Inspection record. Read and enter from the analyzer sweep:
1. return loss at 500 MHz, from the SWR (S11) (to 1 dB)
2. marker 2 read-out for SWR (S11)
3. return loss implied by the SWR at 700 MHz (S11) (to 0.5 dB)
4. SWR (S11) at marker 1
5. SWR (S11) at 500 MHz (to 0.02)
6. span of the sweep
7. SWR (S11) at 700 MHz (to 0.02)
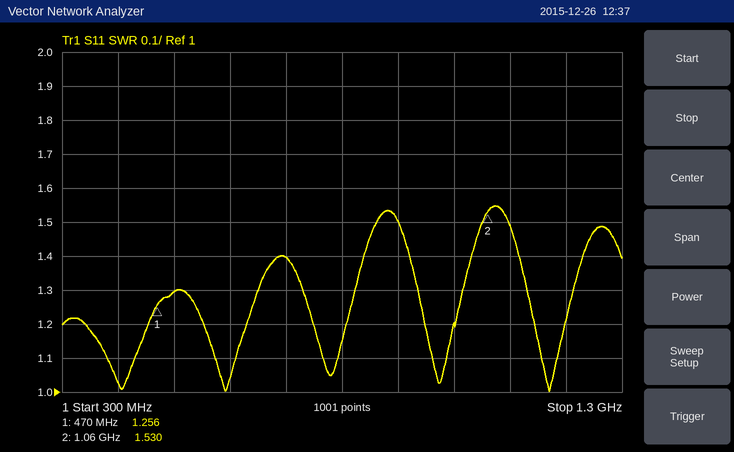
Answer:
18 dB
1.530
15.5 dB
1.256
1.30
1 GHz
1.40
